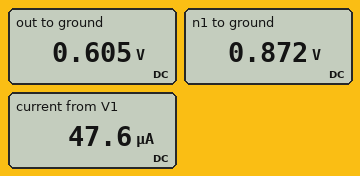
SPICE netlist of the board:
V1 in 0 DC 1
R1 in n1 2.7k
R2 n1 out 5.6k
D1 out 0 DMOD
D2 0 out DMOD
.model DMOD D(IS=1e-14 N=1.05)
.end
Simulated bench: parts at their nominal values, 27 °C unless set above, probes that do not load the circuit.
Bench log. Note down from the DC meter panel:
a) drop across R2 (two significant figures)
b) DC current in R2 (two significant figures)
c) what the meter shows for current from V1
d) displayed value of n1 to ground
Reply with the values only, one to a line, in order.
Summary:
270 mV
48 µA
47.6 µA
0.872 V
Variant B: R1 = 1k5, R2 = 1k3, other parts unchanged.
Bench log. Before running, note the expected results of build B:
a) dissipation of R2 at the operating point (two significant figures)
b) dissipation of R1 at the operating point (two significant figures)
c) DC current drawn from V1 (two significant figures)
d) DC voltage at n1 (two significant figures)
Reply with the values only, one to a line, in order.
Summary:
22 µW
26 µW
130 µA
800 mV
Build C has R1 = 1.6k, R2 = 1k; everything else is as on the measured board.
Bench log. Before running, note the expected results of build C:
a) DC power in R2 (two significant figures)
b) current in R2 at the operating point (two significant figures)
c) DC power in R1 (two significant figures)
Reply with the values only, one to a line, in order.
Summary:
20 µW
140 µA
32 µW
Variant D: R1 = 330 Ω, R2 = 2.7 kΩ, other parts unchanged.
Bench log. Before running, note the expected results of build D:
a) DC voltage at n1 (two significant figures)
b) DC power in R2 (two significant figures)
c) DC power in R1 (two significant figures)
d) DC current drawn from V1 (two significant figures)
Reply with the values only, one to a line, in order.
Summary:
960 mV
40 µW
4.9 µW
120 µA
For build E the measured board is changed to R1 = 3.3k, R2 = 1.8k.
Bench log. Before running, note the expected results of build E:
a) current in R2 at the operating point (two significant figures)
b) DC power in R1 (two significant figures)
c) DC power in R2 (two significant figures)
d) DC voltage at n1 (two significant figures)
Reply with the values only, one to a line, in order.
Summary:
75 µA
19 µW
10 µW
750 mV
